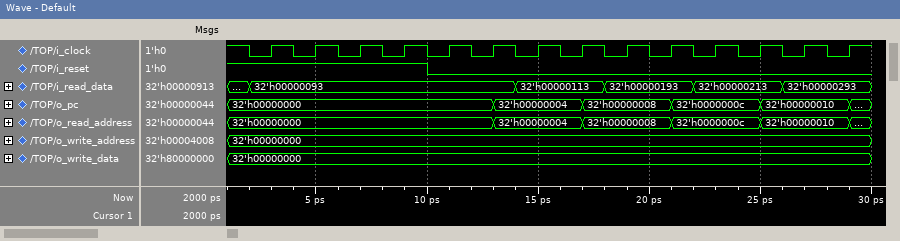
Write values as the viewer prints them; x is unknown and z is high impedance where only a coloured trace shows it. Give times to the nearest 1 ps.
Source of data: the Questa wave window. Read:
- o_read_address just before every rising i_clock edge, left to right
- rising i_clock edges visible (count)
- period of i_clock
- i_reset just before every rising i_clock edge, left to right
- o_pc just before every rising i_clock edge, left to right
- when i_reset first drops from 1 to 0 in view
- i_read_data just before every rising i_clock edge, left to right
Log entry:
32'h00000000, 32'h00000000, 32'h00000000, 32'h00000000, 32'h00000000, 32'h00000000, 32'h00000004, 32'h00000004, 32'h00000008, 32'h00000008, 32'h0000000c, 32'h0000000c, 32'h00000010, 32'h00000010
14
2 ps
1 1 1 1 0 0 0 0 0 0 0 0 0 0
32'h00000000, 32'h00000000, 32'h00000000, 32'h00000000, 32'h00000000, 32'h00000000, 32'h00000004, 32'h00000004, 32'h00000008, 32'h00000008, 32'h0000000c, 32'h0000000c, 32'h00000010, 32'h00000010
10 ps
32'h00000093, 32'h00000093, 32'h00000093, 32'h00000093, 32'h00000093, 32'h00000093, 32'h00000113, 32'h00000113, 32'h00000193, 32'h00000193, 32'h00000213, 32'h00000213, 32'h00000293, 32'h00000293
